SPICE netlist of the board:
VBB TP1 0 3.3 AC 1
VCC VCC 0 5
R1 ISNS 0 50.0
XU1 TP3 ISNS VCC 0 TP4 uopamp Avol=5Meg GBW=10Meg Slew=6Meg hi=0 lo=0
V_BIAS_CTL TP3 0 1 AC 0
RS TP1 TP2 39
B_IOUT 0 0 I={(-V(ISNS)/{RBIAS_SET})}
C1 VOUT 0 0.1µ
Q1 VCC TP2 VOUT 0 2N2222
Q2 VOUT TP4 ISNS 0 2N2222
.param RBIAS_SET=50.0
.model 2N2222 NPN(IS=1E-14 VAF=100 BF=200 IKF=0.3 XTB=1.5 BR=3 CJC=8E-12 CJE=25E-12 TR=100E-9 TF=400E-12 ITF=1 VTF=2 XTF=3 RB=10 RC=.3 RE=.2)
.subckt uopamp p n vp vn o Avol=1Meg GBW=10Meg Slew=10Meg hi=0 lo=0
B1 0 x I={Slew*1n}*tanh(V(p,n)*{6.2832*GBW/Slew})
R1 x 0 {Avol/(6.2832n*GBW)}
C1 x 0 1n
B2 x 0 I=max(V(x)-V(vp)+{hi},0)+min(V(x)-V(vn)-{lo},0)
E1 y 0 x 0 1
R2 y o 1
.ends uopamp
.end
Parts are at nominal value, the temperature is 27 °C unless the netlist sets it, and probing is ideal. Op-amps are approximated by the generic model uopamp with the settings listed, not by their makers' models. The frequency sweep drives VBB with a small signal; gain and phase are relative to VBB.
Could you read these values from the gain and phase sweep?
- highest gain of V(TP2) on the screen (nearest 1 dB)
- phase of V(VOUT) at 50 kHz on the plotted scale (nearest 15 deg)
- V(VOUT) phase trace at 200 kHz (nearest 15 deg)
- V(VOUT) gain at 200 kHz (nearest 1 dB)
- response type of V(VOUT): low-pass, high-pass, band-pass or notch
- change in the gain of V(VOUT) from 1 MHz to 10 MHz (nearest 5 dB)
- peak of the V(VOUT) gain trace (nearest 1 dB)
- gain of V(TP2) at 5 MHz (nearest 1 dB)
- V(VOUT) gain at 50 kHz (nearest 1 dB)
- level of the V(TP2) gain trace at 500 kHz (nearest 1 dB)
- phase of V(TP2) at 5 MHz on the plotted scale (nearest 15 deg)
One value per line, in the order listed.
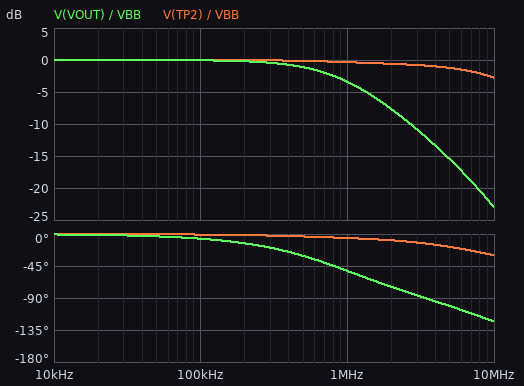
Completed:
0 dB
0 deg
-15 deg
0 dB
low-pass
-20 dB
0 dB
-1 dB
0 dB
0 dB
-15 deg
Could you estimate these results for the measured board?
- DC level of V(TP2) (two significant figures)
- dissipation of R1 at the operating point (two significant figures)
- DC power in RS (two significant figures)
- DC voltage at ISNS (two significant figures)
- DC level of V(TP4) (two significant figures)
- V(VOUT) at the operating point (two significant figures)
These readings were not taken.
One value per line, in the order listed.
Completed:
3.3 V
20 mW
420 nW
1.0 V
1.7 V
2.6 V
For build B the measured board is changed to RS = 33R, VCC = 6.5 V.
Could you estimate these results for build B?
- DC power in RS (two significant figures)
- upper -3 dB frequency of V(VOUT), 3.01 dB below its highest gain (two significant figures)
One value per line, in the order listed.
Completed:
340 nW
930 kHz
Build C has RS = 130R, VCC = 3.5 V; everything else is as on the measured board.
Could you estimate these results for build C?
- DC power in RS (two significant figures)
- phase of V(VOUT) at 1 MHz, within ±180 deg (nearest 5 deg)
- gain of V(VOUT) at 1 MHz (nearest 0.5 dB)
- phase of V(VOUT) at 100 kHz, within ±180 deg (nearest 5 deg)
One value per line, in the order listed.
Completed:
1.4 µW
-65 deg
-4.5 dB
-10 deg
